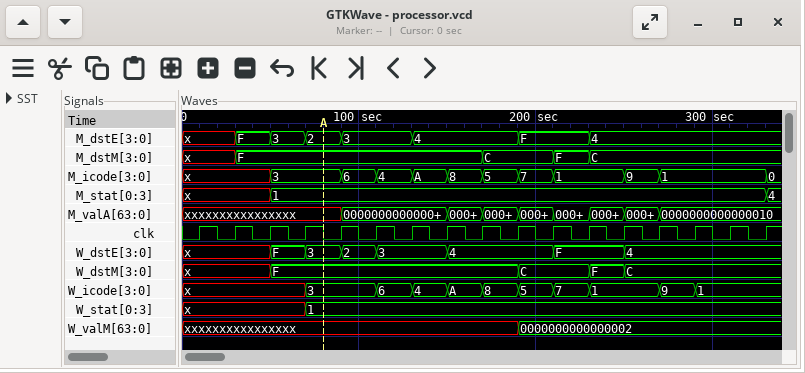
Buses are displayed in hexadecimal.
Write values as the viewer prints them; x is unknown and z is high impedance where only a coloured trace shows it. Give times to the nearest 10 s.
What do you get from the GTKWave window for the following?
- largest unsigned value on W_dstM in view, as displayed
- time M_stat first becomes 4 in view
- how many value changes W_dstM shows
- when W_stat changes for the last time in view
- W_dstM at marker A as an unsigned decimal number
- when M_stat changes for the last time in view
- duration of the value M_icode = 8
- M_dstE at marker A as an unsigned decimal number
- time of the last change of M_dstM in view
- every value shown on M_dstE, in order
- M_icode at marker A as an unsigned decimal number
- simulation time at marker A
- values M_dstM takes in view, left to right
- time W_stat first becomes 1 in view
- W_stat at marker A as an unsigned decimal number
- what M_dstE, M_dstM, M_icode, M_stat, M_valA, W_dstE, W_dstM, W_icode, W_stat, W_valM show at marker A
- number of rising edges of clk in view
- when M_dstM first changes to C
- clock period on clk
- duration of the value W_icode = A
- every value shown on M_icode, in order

F
330 s
4
70 s
15
330 s
20 s
2
230 s
x, F, 3, 2, 3, 4, F, 4
3
80 s
x, F, C, F, C
70 s
1
M_dstE=2, M_dstM=F, M_icode=3, M_stat=1, M_valA=xxxxxxxxxxxxxxxx, W_dstE=3, W_dstM=F, W_icode=3, W_stat=1, W_valM=xxxxxxxxxxxxxxxx
17
170 s
20 s
20 s
x, 3, 6, 4, A, 8, 5, 7, 1, 9, 1, 0
